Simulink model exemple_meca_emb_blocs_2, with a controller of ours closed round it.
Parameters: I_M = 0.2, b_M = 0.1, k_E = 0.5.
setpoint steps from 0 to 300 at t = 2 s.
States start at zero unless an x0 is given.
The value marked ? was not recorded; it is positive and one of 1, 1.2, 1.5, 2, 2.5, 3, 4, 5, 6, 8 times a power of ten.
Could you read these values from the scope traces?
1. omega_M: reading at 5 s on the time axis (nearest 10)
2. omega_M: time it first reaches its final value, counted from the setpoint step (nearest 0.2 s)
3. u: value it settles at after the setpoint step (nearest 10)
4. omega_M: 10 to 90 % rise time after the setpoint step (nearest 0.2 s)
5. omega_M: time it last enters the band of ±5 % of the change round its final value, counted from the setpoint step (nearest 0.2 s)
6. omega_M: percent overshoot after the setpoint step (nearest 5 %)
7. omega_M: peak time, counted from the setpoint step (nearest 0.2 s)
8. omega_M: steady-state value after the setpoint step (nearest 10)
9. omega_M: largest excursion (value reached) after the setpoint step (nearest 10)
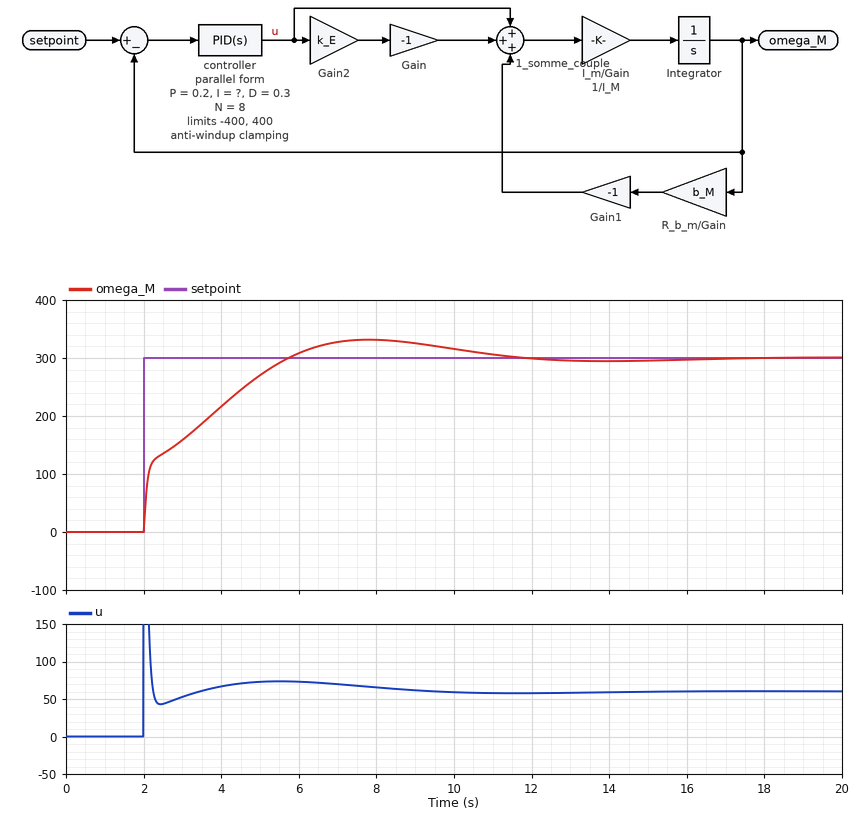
270
3.8 s
60
3.0 s
8.0 s
10 %
5.8 s
300
330
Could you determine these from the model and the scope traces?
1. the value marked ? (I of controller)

0.25
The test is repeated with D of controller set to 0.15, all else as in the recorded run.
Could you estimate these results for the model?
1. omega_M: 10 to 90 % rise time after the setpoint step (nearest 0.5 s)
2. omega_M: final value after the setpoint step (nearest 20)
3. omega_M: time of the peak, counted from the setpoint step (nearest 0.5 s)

2.5 s
300
5.0 s
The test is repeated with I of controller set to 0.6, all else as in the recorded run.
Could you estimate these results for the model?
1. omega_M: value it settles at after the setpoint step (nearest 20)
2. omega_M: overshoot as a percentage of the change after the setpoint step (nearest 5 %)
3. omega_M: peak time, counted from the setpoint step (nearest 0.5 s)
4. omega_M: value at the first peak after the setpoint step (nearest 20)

300
20 %
3.5 s
360
